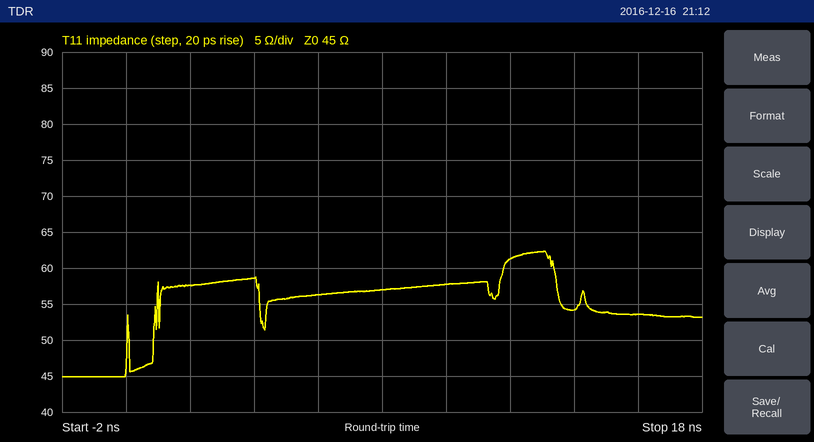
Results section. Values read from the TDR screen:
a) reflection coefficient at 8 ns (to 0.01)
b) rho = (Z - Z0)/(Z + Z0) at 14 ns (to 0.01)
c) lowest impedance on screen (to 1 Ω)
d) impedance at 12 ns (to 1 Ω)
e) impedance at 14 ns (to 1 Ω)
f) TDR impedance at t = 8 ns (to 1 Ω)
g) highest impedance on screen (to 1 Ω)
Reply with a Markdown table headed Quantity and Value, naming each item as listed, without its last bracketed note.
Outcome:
| Quantity | Value |
|---|---|
| reflection coefficient at 8 ns | +0.12 |
| rho = (Z - Z0)/(Z + Z0) at 14 ns | +0.09 |
| lowest impedance on screen | 45 Ω |
| impedance at 12 ns | 61 Ω |
| impedance at 14 ns | 54 Ω |
| TDR impedance at t = 8 ns | 57 Ω |
| highest impedance on screen | 62 Ω |
